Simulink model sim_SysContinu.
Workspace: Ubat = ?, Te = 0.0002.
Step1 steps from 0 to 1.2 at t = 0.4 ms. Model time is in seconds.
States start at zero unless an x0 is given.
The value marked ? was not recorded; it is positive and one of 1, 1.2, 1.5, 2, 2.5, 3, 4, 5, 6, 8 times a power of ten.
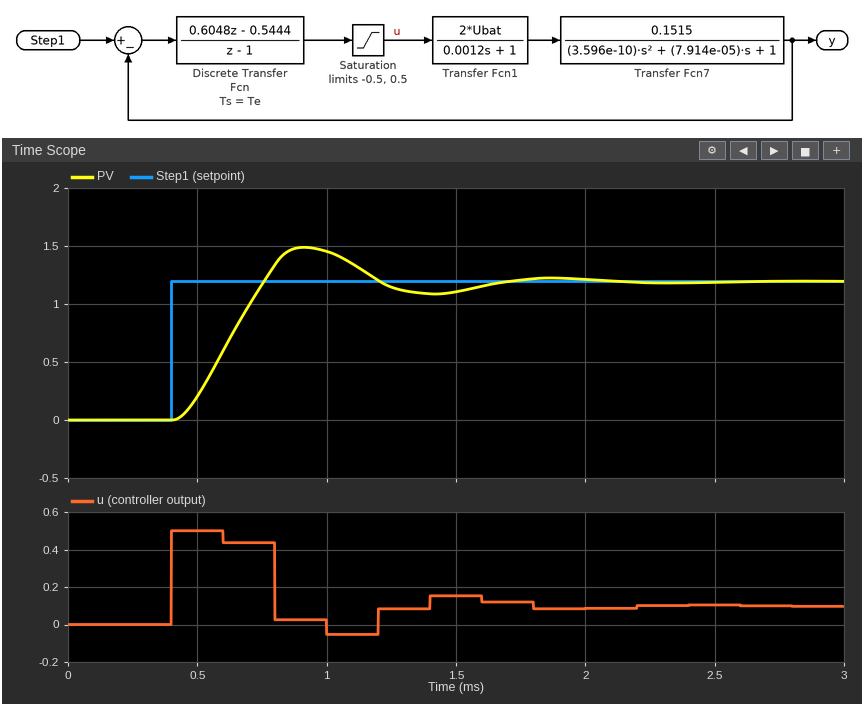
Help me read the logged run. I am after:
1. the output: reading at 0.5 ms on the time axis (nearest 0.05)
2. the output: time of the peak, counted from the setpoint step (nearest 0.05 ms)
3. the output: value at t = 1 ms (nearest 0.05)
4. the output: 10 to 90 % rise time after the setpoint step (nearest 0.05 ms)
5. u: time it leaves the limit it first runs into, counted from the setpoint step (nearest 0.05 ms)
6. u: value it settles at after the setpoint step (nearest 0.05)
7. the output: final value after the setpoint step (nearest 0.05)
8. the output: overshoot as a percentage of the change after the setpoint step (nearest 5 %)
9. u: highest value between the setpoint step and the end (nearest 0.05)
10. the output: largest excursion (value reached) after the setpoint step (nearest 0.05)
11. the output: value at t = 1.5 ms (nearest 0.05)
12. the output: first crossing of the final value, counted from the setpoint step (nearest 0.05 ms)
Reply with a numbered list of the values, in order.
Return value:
1. 0.20
2. 0.50 ms
3. 1.45
4. 0.25 ms
5. 0.20 ms
6. 0.10
7. 1.20
8. 25 %
9. 0.50
10. 1.50
11. 1.10
12. 0.35 ms
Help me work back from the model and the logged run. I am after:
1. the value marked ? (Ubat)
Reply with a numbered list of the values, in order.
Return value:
1. 40
